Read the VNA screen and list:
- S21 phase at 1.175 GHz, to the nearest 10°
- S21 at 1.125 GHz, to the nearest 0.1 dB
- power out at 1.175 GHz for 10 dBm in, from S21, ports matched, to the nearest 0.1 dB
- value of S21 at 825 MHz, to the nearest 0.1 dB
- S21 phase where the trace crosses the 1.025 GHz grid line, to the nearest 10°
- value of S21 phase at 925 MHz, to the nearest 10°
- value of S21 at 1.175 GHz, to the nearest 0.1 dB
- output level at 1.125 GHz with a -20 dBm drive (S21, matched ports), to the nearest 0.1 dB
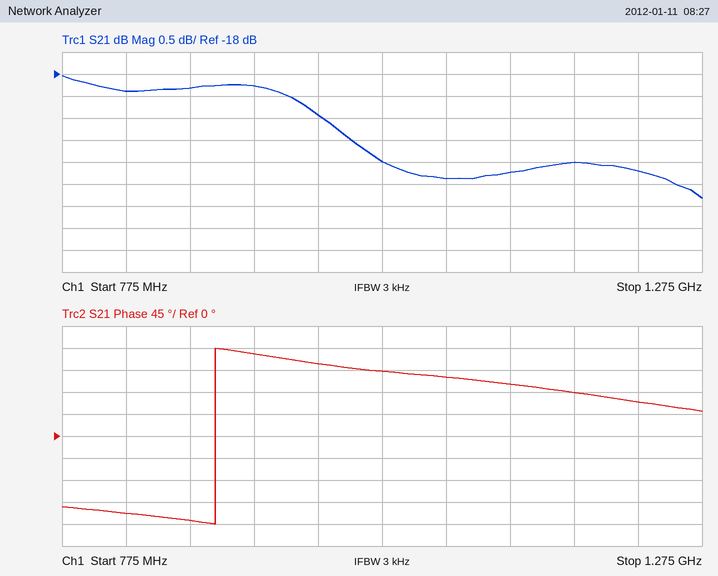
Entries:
90°
-20.2 dB
-10.0 dBm
-18.4 dB
130°
170°
-20.0 dB
-40.2 dBm
